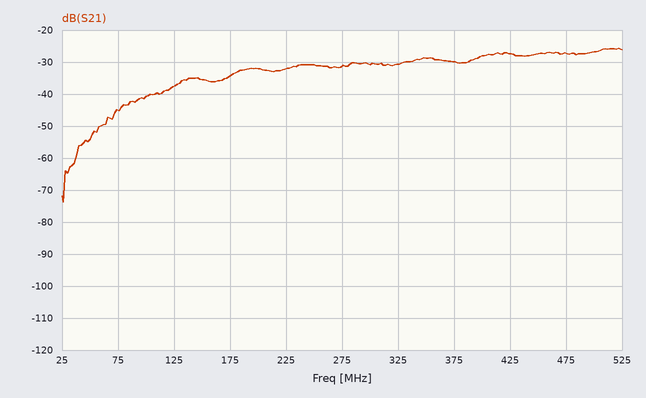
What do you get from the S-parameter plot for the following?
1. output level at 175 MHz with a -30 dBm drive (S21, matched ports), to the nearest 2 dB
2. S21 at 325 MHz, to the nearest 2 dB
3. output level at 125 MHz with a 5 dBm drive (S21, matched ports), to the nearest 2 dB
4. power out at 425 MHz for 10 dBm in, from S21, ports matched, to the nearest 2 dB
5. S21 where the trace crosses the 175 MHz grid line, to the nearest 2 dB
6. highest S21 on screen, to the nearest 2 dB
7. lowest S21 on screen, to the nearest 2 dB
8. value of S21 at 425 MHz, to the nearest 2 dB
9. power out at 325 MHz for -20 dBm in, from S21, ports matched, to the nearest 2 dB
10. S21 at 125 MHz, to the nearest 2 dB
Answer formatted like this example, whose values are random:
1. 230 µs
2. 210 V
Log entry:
1. -64 dBm
2. -30 dB
3. -32 dBm
4. -18 dBm
5. -34 dB
6. -26 dB
7. -74 dB
8. -28 dB
9. -50 dBm
10. -38 dB
